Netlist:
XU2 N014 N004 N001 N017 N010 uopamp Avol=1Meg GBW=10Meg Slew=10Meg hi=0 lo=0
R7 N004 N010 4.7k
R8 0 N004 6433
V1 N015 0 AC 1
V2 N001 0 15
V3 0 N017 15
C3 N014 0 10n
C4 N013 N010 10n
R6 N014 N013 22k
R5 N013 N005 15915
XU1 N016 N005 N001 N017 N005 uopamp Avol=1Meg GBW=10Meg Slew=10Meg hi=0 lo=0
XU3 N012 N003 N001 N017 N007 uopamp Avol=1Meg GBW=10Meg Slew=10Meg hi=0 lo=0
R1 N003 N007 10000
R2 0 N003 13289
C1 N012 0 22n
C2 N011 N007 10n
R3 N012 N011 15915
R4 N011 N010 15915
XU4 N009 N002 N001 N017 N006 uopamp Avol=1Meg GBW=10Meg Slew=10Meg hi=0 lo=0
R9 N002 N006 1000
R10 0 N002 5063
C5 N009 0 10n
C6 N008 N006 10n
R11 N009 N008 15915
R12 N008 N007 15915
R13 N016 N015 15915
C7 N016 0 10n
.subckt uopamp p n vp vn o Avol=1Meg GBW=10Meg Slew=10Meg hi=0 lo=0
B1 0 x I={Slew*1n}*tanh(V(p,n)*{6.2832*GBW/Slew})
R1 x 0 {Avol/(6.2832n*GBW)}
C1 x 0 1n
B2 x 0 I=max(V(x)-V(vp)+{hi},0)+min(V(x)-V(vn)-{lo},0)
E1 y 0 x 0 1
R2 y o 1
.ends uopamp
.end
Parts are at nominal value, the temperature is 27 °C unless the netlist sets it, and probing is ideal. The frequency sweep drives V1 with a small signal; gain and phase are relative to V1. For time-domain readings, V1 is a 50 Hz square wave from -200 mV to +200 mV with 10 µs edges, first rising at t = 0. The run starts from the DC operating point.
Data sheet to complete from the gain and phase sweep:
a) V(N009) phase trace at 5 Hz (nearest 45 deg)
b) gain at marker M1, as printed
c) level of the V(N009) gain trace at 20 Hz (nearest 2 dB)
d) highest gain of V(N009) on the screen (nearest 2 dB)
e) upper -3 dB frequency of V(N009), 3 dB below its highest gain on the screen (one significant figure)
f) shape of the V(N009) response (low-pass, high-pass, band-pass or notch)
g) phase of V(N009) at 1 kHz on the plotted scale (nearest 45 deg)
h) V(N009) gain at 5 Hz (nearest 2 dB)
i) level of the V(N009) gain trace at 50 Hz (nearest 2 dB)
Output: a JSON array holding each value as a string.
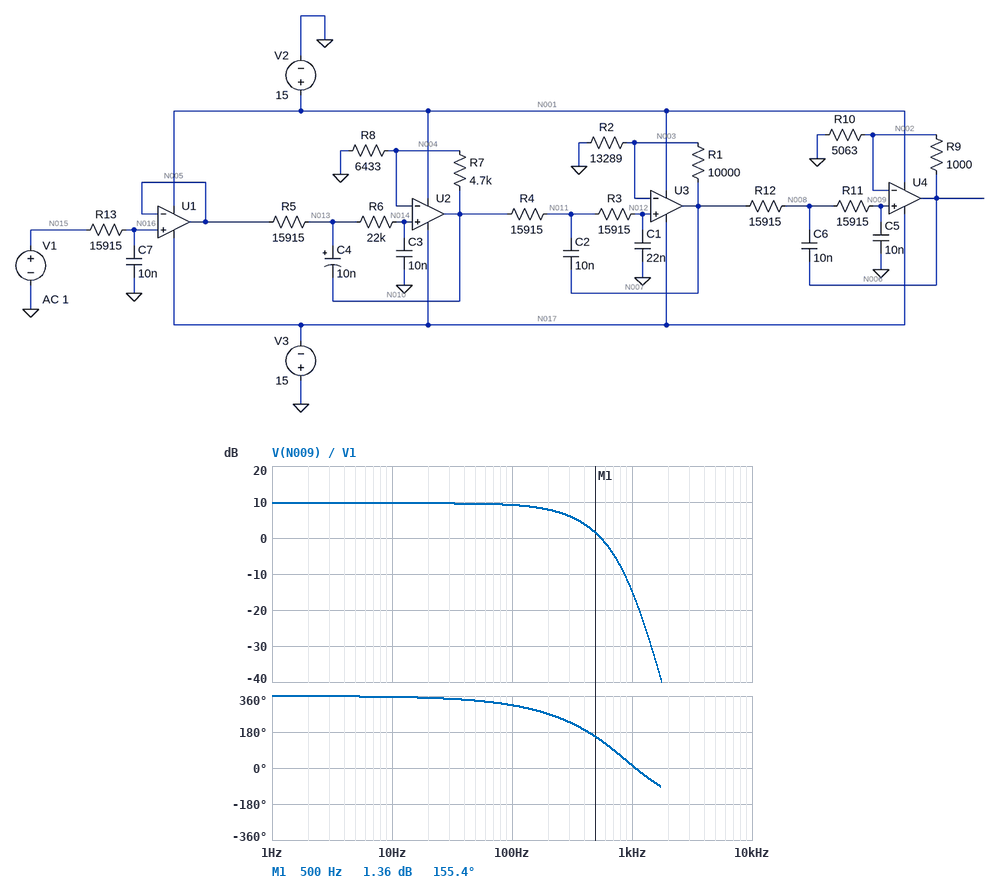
["360 deg", "1.36 dB", "10 dB", "10 dB", "300 Hz", "low-pass", "0 deg", "10 dB", "10 dB"]
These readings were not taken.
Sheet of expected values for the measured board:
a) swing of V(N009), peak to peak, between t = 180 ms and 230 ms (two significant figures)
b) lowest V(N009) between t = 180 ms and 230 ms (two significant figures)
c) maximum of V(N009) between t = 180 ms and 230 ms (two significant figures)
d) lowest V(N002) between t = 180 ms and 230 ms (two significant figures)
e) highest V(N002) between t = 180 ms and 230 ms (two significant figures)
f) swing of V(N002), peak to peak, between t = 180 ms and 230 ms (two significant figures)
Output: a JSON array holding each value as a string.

["1.2 V", "-610 mV", "610 mV", "-610 mV", "610 mV", "1.2 V"]
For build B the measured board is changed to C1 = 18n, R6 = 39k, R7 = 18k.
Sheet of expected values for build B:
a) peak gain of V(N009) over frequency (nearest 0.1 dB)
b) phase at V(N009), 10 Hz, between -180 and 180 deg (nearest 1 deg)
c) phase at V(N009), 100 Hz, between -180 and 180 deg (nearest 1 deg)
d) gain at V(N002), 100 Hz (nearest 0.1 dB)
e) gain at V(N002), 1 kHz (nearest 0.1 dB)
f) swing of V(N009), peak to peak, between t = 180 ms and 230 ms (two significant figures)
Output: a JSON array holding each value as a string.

["16.5 dB", "-4 deg", "-36 deg", "16.4 dB", "-5.1 dB", "3.3 V"]
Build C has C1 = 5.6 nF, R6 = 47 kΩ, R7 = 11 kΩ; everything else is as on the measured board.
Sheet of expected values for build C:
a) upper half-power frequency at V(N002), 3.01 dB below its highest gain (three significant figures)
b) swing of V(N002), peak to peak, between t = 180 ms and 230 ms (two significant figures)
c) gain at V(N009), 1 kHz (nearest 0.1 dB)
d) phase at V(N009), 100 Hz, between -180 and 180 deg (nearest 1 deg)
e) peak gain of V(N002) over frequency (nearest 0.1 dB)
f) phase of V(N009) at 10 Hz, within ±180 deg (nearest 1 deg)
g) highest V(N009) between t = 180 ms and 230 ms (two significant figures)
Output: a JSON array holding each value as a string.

["533 Hz", "2.1 V", "0.8 dB", "-31 deg", "13.5 dB", "-3 deg", "1.0 V"]
